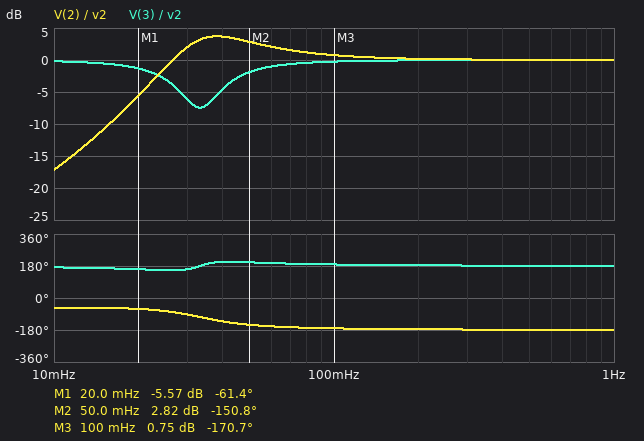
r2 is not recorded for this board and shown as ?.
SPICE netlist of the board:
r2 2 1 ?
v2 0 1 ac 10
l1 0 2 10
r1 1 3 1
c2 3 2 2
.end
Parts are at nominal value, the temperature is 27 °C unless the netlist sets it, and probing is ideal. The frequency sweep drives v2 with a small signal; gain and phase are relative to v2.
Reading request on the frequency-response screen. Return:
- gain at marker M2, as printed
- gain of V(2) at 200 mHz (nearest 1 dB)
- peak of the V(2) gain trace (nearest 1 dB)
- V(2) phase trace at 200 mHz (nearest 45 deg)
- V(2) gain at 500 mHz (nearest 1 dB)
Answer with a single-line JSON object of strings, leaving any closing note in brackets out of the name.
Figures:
{"gain at marker M2, as printed": "2.82 dB", "gain of V(2) at 200 mHz": "0 dB", "peak of the V(2) gain trace": "4 dB", "V(2) phase trace at 200 mHz": "-180 deg", "V(2) gain at 500 mHz": "0 dB"}
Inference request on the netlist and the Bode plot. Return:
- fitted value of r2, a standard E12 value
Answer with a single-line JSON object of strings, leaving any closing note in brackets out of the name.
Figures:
{"fitted value of r2, a standard E12 value": "6.8 Ω"}
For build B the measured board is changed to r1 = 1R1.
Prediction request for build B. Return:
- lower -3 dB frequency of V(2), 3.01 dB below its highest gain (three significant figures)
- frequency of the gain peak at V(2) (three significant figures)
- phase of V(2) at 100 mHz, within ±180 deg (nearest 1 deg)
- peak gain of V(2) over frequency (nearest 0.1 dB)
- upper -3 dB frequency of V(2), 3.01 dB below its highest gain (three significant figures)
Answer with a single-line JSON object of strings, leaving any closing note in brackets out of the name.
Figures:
{"lower -3 dB frequency of V(2), 3.01 dB below its highest gain": "27.3 mHz", "frequency of the gain peak at V(2)": "38.6 mHz", "phase of V(2) at 100 mHz, within ±180 deg": "-170 deg", "peak gain of V(2) over frequency": "3.3 dB", "upper -3 dB frequency of V(2), 3.01 dB below its highest gain": "150 mHz"}
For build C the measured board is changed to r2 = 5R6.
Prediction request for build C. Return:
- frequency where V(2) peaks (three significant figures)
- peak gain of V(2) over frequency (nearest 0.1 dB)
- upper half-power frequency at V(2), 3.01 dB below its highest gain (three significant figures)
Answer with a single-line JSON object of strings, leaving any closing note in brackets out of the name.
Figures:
{"frequency where V(2) peaks": "38.4 mHz", "peak gain of V(2) over frequency": "3.3 dB", "upper half-power frequency at V(2), 3.01 dB below its highest gain": "164 mHz"}
